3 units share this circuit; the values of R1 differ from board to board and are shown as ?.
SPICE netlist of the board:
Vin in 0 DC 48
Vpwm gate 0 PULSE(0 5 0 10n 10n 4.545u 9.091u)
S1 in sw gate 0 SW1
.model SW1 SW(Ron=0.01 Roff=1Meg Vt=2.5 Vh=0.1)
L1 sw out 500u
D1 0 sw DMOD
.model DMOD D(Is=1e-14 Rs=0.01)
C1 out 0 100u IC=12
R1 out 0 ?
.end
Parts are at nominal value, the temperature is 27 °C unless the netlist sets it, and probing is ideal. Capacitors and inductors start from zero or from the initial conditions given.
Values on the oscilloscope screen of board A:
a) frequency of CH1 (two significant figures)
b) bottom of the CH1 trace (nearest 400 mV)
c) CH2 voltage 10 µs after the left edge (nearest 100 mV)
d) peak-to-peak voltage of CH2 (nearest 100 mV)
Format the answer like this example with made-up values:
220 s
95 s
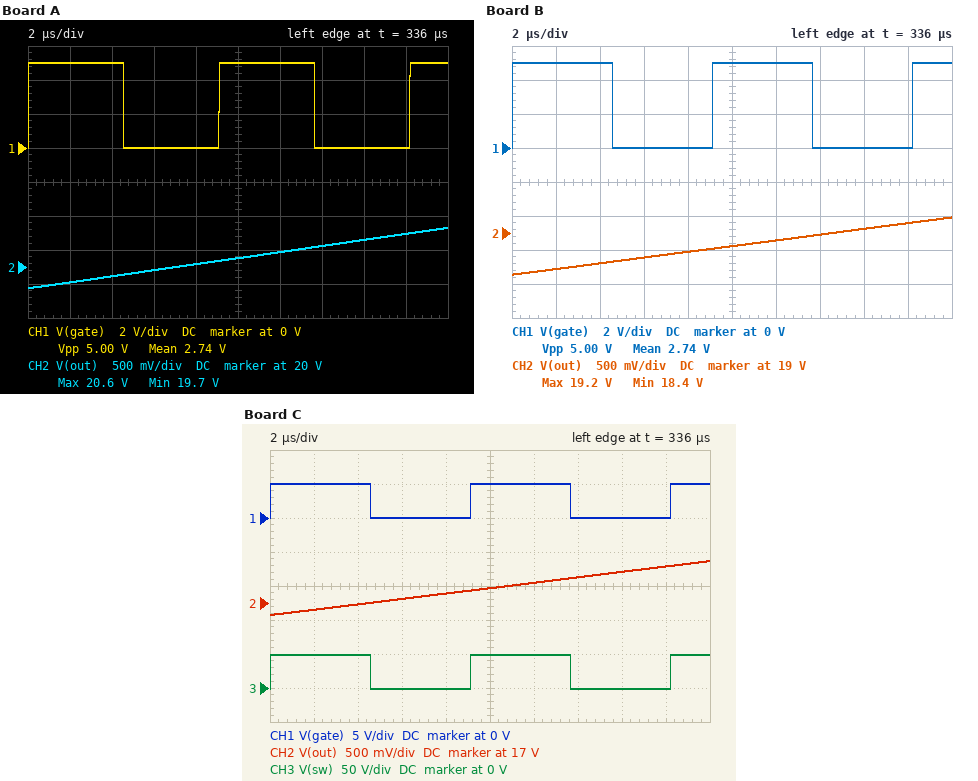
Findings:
110 kHz
0 V
20.1 V
900 mV
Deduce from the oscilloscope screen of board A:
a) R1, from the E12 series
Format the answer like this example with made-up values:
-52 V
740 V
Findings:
10 Ω
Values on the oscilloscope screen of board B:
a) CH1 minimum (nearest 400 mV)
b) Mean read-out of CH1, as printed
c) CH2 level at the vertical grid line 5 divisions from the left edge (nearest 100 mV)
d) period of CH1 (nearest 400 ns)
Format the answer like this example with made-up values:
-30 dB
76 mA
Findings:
0 V
2.74 V
18.8 V
9.2 µs
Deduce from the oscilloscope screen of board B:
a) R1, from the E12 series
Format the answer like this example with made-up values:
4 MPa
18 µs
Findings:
6.8 Ω
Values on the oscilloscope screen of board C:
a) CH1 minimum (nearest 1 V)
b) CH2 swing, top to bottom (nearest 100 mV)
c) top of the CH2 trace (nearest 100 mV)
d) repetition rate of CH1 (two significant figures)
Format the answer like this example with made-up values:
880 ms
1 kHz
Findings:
0 V
800 mV
17.6 V
110 kHz
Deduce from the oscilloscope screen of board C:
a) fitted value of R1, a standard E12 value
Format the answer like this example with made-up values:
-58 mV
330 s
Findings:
4.7 Ω
